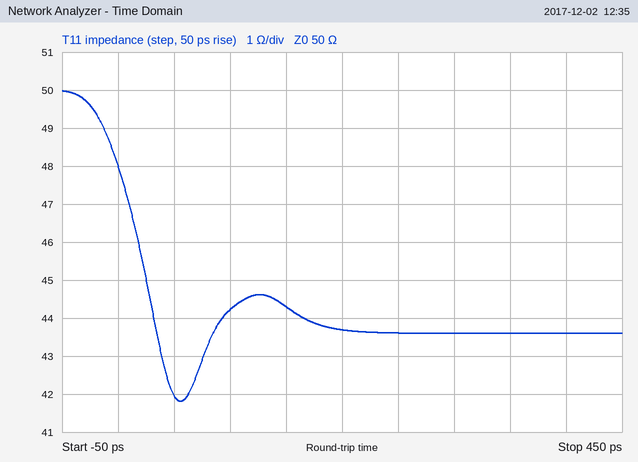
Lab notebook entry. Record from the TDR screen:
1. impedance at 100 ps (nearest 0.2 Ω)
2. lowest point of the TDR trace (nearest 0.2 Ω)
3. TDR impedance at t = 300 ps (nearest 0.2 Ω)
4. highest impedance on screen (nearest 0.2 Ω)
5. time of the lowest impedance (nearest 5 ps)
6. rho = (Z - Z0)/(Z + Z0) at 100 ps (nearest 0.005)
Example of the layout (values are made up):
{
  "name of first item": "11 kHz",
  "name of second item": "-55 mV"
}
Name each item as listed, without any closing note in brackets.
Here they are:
{
  "impedance at 100 ps": "44.2 Ω",
  "lowest point of the TDR trace": "41.8 Ω",
  "TDR impedance at t = 300 ps": "43.6 Ω",
  "highest impedance on screen": "50.0 Ω",
  "time of the lowest impedance": "55 ps",
  "rho = (Z - Z0)/(Z + Z0) at 100 ps": "-0.060"
}
